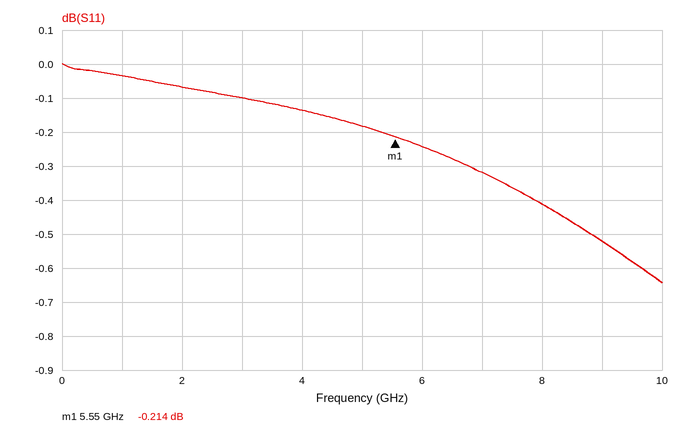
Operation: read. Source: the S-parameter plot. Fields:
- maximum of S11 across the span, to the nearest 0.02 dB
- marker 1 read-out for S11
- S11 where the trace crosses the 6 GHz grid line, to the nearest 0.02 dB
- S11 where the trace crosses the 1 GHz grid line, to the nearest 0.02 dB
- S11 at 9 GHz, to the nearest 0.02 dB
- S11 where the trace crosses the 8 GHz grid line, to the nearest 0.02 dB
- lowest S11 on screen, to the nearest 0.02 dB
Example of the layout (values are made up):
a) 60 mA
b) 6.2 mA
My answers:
a) 0.00 dB
b) -0.214 dB
c) -0.24 dB
d) -0.04 dB
e) -0.52 dB
f) -0.42 dB
g) -0.64 dB
